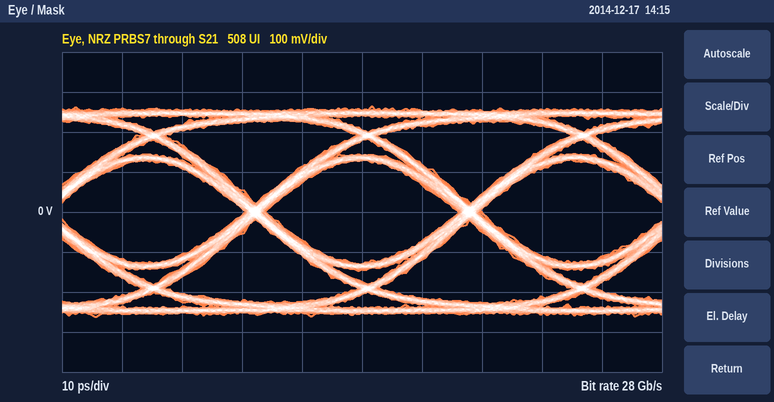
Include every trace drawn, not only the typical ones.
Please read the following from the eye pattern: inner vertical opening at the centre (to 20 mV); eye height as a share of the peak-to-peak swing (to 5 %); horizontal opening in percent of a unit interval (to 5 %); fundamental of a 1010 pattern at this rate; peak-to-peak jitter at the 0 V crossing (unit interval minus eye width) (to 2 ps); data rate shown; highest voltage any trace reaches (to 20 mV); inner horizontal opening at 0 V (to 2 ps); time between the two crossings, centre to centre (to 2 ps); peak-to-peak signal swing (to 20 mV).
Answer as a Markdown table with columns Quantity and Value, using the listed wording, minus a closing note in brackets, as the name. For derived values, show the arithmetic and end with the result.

| Quantity | Value |
|---|---|
| inner vertical opening at the centre | 260 mV |
| eye height as a share of the peak-to-peak swing | 260 mV / 520 mV ≈ 50 % |
| horizontal opening in percent of a unit interval | 32 ps / 36 ps ≈ 88.9 %, so 90 % to the nearest 5 % |
| fundamental of a 1010 pattern at this rate | 14 GHz |
| peak-to-peak jitter at the 0 V crossing (unit interval minus eye width) | 4 ps |
| data rate shown | 28 Gb/s |
| highest voltage any trace reaches | 260 mV |
| inner horizontal opening at 0 V | 32 ps |
| time between the two crossings, centre to centre | 36 ps |
| peak-to-peak signal swing | 520 mV |
